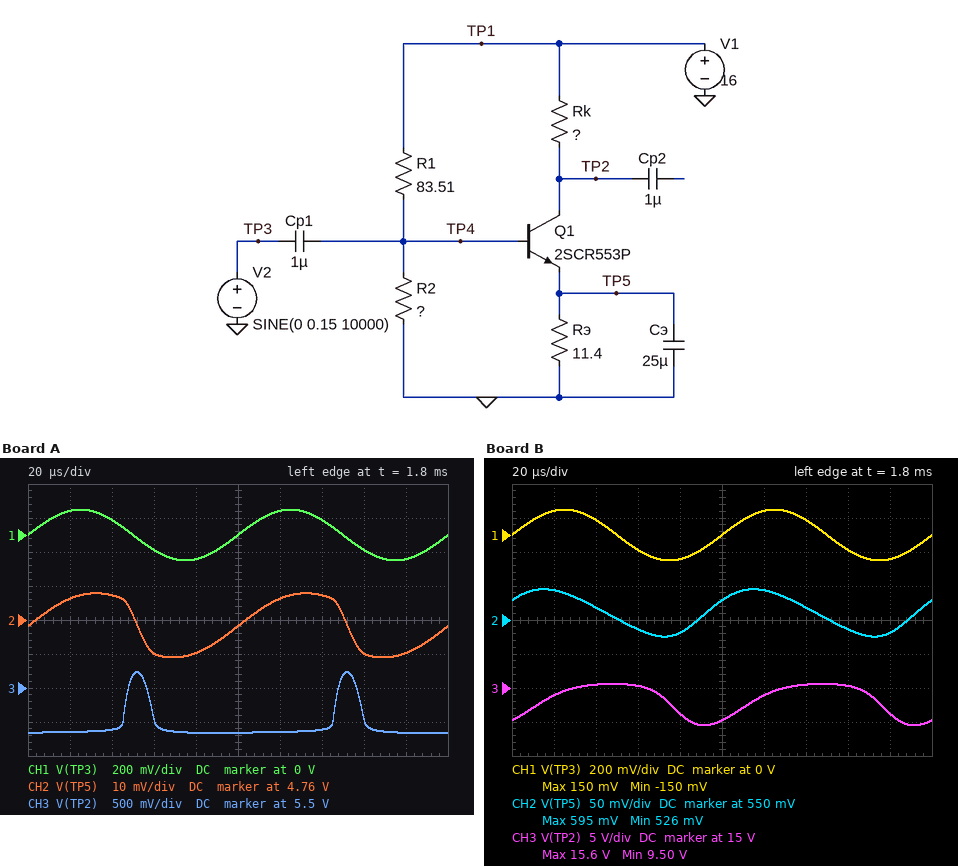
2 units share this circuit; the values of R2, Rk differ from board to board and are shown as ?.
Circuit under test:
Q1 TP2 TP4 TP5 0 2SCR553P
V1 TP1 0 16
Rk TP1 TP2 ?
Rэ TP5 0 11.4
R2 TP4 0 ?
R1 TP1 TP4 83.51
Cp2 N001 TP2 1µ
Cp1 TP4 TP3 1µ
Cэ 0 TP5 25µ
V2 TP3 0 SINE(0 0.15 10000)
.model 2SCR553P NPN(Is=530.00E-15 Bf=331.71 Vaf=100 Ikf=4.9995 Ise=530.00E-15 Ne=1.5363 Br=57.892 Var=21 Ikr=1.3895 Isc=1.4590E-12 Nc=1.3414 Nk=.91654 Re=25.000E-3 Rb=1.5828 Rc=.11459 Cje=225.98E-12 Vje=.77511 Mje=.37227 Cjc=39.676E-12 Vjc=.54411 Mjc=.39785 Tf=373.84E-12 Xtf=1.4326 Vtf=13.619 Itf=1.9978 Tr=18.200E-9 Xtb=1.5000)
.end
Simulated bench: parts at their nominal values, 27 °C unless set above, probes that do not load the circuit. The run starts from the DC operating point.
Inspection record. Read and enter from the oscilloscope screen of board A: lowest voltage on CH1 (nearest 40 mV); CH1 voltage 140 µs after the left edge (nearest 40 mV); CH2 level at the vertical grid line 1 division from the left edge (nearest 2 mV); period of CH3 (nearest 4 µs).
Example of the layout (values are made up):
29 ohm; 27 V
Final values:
-160 mV; 80 mV; 4.766 V; 100 µs
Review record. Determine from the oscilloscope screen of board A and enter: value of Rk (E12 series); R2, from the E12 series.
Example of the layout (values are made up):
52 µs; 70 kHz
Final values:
27 Ω; 47 Ω
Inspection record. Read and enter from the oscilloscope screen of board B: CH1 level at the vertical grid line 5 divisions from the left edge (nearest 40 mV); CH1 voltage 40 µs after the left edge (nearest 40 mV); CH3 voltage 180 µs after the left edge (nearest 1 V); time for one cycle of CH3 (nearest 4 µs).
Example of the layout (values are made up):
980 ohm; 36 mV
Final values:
0 V; 80 mV; 11 V; 100 µs
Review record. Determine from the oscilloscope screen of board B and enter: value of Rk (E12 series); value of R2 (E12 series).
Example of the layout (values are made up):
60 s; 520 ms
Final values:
56 Ω; 6.8 Ω
